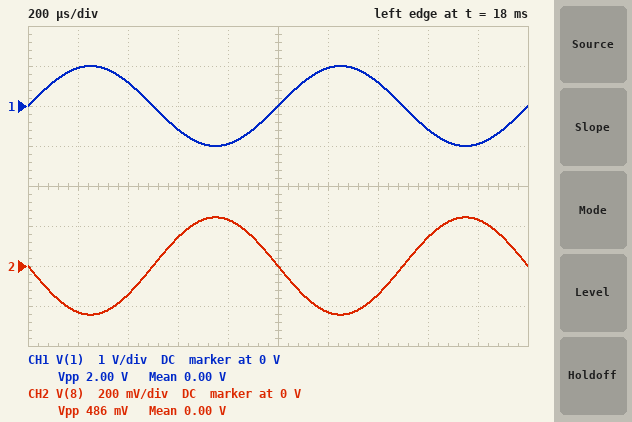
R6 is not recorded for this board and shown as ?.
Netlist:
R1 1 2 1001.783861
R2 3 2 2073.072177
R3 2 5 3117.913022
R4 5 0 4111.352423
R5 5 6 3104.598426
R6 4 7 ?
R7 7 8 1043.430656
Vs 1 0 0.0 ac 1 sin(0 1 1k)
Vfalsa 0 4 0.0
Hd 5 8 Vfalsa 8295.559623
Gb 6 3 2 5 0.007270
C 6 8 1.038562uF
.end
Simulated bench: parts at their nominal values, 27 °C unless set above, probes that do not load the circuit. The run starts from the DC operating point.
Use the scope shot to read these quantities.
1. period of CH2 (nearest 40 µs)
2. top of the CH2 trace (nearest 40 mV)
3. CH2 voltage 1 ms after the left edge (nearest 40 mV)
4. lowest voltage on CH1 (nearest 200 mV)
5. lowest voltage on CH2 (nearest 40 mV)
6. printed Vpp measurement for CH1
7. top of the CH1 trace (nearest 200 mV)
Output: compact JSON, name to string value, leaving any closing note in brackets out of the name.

{"period of CH2": "1.00 ms", "top of the CH2 trace": "240 mV", "CH2 voltage 1 ms after the left edge": "0 V", "lowest voltage on CH1": "-1.0 V", "lowest voltage on CH2": "-240 mV", "printed Vpp measurement for CH1": "2.00 V", "top of the CH1 trace": "1.0 V"}
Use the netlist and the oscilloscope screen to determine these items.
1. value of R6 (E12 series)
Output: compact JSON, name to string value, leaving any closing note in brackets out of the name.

{"value of R6": "680 Ω"}
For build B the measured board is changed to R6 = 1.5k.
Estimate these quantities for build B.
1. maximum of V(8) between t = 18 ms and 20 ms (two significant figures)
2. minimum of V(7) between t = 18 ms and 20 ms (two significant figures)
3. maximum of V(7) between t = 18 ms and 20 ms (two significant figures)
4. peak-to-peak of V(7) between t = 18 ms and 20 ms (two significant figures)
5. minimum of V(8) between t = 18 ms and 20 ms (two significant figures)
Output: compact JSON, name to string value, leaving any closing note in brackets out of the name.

{"maximum of V(8) between t = 18 ms and 20 ms": "420 mV", "minimum of V(7) between t = 18 ms and 20 ms": "-250 mV", "maximum of V(7) between t = 18 ms and 20 ms": "250 mV", "peak-to-peak of V(7) between t = 18 ms and 20 ms": "490 mV", "minimum of V(8) between t = 18 ms and 20 ms": "-420 mV"}
